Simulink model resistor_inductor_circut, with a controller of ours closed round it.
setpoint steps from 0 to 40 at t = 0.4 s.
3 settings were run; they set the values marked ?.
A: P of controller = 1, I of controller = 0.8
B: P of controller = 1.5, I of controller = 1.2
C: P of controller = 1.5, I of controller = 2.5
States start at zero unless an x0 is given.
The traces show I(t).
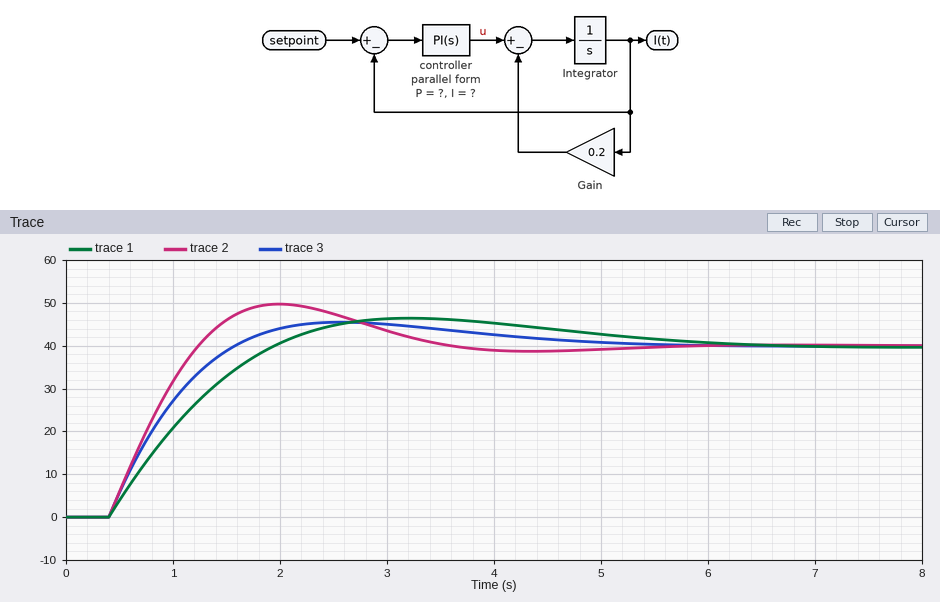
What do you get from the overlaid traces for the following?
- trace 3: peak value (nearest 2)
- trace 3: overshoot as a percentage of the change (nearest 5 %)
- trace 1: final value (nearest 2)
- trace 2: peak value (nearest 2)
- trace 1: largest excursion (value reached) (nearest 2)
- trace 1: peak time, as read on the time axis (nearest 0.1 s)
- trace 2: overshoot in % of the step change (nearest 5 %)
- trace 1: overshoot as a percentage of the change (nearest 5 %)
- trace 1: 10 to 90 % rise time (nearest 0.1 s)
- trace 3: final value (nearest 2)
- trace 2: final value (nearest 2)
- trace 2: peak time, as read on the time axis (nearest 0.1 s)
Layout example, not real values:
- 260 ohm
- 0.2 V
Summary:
- 46
- 15 %
- 40
- 50
- 46
- 3.2 s
- 25 %
- 15 %
- 1.2 s
- 40
- 40
- 2.0 s
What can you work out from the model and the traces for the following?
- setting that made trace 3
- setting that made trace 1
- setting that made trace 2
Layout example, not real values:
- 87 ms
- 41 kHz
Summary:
- B
- A
- C
